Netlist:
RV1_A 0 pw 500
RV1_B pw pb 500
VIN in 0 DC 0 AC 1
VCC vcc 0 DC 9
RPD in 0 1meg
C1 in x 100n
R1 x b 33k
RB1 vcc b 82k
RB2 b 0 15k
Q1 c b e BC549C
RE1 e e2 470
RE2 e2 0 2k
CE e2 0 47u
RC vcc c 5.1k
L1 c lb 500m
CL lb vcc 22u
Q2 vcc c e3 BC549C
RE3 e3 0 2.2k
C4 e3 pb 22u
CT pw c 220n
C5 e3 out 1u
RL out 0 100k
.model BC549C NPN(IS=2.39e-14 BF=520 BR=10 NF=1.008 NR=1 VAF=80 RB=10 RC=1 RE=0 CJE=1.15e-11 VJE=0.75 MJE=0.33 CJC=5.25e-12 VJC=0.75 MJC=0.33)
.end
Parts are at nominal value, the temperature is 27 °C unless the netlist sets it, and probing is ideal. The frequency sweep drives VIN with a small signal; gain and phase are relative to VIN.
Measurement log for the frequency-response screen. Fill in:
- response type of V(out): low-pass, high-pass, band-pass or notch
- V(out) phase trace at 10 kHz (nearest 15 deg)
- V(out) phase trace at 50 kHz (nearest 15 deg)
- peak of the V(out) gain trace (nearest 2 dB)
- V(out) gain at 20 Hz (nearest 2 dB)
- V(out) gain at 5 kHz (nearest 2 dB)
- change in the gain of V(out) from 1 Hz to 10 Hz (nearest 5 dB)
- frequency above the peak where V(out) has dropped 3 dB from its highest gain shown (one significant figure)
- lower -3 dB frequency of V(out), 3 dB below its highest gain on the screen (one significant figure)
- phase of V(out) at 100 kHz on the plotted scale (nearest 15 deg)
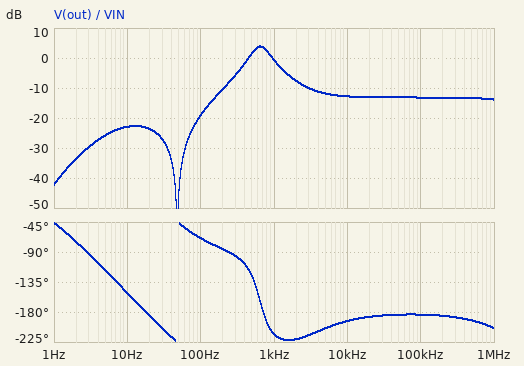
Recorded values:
band-pass
-195 deg
-180 deg
4 dB
-24 dB
-12 dB
20 dB
900 Hz
500 Hz
-180 deg
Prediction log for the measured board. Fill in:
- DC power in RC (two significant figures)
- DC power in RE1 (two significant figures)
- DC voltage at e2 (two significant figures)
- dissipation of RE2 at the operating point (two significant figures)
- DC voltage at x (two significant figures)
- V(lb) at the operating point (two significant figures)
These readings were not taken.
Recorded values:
520 µW
47 µW
630 mV
200 µW
1.4 V
7.4 V
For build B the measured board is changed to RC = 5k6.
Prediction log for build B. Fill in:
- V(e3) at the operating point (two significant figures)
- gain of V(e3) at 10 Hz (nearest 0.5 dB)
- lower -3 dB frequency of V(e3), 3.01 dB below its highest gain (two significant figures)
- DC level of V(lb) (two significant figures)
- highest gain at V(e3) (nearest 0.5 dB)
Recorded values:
6.5 V
-23.0 dB
490 Hz
7.2 V
4.5 dB
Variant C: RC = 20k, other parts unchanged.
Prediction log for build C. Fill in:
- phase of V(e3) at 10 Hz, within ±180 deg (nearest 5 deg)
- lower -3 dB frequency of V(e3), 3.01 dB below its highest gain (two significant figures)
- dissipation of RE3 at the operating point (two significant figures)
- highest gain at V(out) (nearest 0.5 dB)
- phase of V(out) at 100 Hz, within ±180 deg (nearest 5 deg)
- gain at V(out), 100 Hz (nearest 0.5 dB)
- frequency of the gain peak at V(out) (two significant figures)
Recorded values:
-165 deg
560 Hz
1.9 mW
9.0 dB
-65 deg
-19.5 dB
660 Hz
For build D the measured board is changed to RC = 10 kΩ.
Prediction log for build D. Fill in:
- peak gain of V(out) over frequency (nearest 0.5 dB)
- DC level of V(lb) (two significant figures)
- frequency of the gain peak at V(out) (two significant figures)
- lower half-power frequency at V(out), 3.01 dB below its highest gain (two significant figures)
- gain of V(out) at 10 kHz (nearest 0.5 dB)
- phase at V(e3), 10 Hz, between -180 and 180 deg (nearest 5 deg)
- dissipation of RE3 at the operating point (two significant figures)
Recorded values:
7.0 dB
5.8 V
660 Hz
530 Hz
-12.5 dB
-165 deg
12 mW
